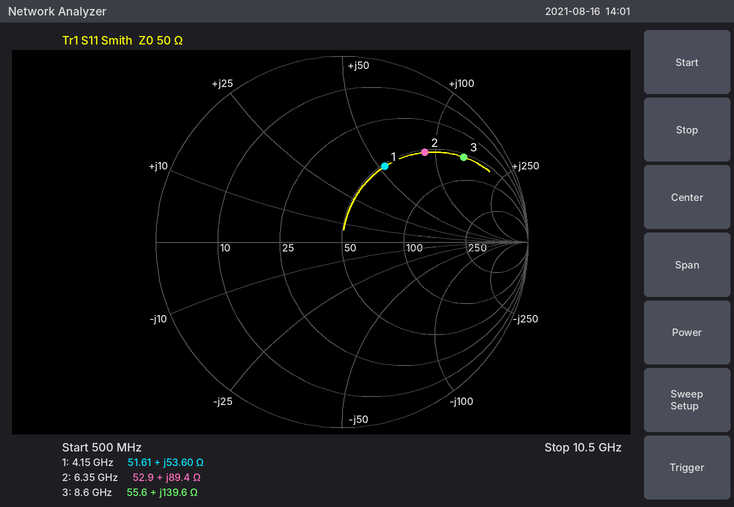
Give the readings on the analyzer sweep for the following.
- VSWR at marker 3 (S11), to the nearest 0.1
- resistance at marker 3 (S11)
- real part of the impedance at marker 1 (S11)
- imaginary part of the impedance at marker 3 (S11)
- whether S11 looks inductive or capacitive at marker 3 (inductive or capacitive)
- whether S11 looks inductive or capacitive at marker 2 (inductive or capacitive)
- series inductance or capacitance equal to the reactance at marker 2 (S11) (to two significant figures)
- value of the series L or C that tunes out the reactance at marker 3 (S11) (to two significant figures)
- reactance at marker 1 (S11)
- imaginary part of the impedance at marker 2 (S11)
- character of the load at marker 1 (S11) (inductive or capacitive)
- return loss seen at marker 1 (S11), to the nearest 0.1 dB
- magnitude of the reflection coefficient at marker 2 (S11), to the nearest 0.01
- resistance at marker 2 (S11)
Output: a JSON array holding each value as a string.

["8.9", "55.6 Ω", "51.61 Ω", "+139.6 Ω", "inductive", "inductive", "2.2 nH", "130 fF", "+53.60 Ω", "+89.4 Ω", "inductive", "6.6 dB", "0.66", "52.9 Ω"]
